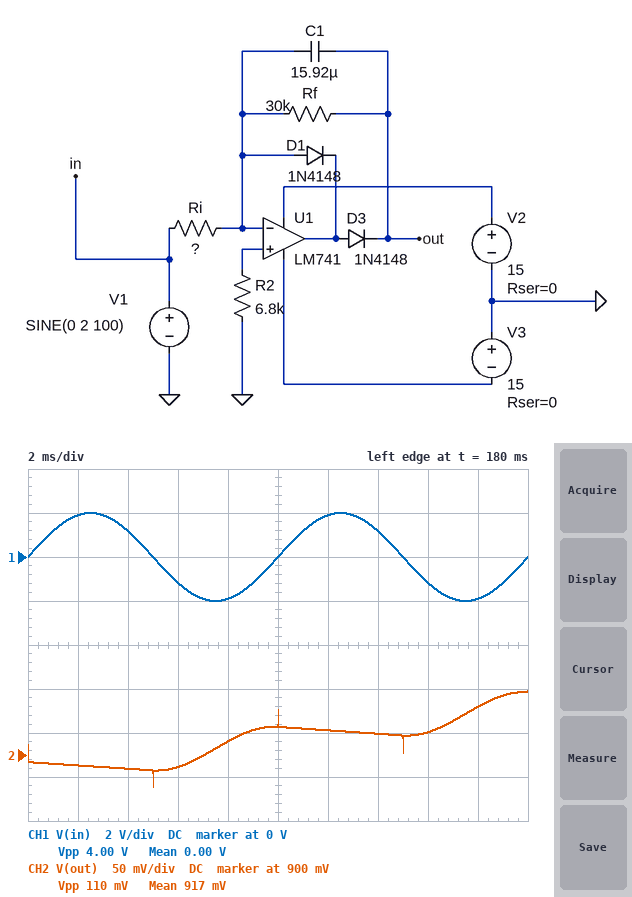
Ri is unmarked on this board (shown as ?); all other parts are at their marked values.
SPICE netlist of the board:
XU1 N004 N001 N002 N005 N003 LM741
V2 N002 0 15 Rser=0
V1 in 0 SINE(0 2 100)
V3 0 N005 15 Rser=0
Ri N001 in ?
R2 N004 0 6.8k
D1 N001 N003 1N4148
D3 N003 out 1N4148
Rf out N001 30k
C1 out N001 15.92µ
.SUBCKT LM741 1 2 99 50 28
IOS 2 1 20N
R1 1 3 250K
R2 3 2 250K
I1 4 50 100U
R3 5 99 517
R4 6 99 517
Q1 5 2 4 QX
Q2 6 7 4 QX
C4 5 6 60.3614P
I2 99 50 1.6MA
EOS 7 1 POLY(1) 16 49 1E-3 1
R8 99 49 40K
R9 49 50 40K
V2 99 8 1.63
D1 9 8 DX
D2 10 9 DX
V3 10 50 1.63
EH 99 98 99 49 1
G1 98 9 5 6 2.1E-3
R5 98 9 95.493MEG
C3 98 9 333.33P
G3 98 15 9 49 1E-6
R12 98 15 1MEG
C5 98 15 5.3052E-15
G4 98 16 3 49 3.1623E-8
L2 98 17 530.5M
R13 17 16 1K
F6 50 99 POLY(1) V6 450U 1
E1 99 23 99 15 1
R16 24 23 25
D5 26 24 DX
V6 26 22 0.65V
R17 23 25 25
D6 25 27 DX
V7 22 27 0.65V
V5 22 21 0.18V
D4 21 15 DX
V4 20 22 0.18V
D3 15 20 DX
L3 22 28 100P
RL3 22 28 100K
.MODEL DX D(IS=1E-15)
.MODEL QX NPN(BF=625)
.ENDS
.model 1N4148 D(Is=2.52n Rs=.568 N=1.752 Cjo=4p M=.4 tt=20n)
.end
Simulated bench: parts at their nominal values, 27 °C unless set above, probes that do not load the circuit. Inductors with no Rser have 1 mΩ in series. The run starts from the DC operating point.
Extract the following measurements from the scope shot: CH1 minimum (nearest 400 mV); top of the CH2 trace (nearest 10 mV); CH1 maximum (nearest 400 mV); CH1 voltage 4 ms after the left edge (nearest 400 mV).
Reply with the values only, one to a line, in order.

-2.0 V
970 mV
2.0 V
1.2 V
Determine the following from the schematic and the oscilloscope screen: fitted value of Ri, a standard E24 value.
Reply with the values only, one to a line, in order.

6.8 kΩ
